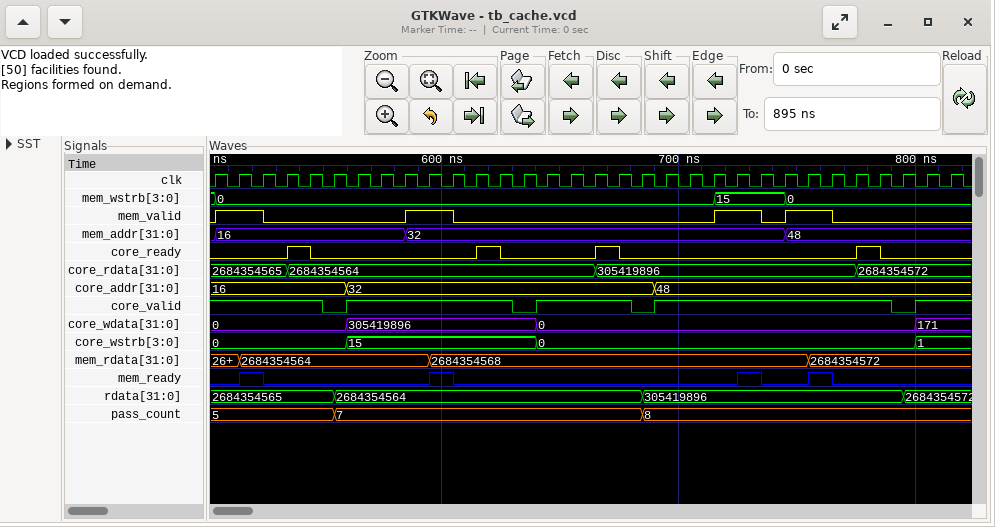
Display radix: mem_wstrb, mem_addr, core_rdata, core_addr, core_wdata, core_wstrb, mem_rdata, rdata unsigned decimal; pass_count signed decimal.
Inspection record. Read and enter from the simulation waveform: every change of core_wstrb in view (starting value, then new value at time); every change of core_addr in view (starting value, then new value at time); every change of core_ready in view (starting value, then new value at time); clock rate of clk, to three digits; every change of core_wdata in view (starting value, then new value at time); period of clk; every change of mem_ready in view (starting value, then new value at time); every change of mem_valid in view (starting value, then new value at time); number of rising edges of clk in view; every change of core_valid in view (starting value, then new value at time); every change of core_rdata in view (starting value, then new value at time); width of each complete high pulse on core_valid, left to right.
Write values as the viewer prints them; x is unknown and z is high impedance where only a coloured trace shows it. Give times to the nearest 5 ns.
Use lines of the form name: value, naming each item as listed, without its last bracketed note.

every change of core_wstrb in view: 0, 15 at 560 ns, 0 at 640 ns, 1 at 800 ns
every change of core_addr in view: 16, 32 at 560 ns, 48 at 690 ns
every change of core_ready in view: 0, 1 at 535 ns, 0 at 545 ns, 1 at 615 ns, 0 at 625 ns, 1 at 665 ns, 0 at 675 ns, 1 at 775 ns, 0 at 785 ns
clock rate of clk, to three digits: 100 MHz
every change of core_wdata in view: 0, 305419896 at 560 ns, 0 at 640 ns, 171 at 800 ns
period of clk: 10 ns
every change of mem_ready in view: 0, 1 at 515 ns, 0 at 525 ns, 1 at 595 ns, 0 at 605 ns, 1 at 725 ns, 0 at 735 ns, 1 at 755 ns, 0 at 765 ns
every change of mem_valid in view: 0, 1 at 505 ns, 0 at 525 ns, 1 at 585 ns, 0 at 605 ns, 1 at 715 ns, 0 at 735 ns, 1 at 745 ns, 0 at 765 ns
number of rising edges of clk in view: 32
every change of core_valid in view: 1, 0 at 550 ns, 1 at 560 ns, 0 at 630 ns, 1 at 640 ns, 0 at 680 ns, 1 at 690 ns, 0 at 790 ns, 1 at 800 ns
every change of core_rdata in view: 2684354565, 2684354564 at 535 ns, 305419896 at 665 ns, 2684354572 at 775 ns
width of each complete high pulse on core_valid, left to right: 70 ns, 40 ns, 100 ns
